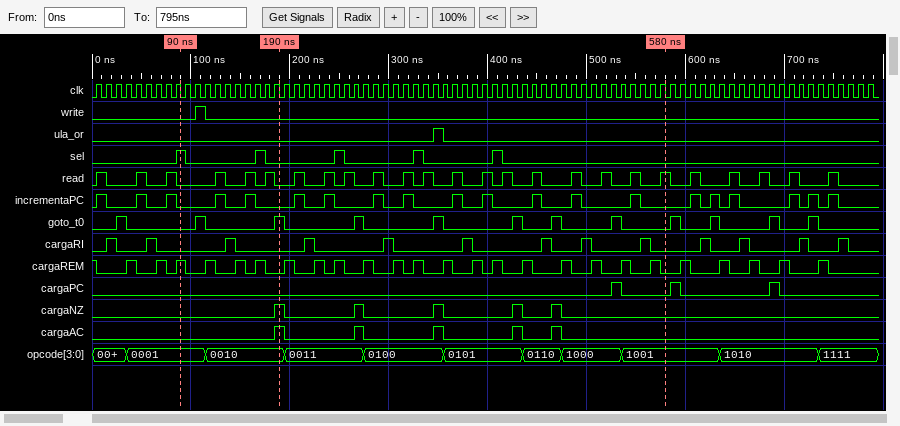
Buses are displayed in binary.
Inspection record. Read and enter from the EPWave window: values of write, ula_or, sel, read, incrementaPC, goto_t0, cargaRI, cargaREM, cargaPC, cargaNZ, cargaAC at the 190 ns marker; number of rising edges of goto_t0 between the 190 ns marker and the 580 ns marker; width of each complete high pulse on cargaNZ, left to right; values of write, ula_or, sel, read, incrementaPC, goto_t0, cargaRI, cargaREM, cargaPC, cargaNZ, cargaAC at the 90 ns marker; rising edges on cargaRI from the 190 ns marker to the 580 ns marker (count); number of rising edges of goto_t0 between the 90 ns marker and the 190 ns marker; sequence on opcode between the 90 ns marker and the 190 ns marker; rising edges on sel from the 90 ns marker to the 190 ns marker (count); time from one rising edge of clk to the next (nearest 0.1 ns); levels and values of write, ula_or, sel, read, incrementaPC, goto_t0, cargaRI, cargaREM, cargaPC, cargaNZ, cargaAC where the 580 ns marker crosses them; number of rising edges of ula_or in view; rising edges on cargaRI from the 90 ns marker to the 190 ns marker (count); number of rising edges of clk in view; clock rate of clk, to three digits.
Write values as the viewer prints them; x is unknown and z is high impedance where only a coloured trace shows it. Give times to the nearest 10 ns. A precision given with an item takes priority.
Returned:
write=0, ula_or=0, sel=0, read=0, incrementaPC=0, goto_t0=1, cargaRI=0, cargaREM=0, cargaPC=0, cargaNZ=1, cargaAC=1
5
10 ns, 10 ns, 10 ns, 10 ns, 10 ns
write=0, ula_or=0, sel=1, read=0, incrementaPC=0, goto_t0=0, cargaRI=0, cargaREM=1, cargaPC=0, cargaNZ=0, cargaAC=0
6
2
0001, 0010
1
10 ns
write=0, ula_or=0, sel=0, read=1, incrementaPC=0, goto_t0=0, cargaRI=0, cargaREM=0, cargaPC=0, cargaNZ=0, cargaAC=0
1
1
79
100 MHz
